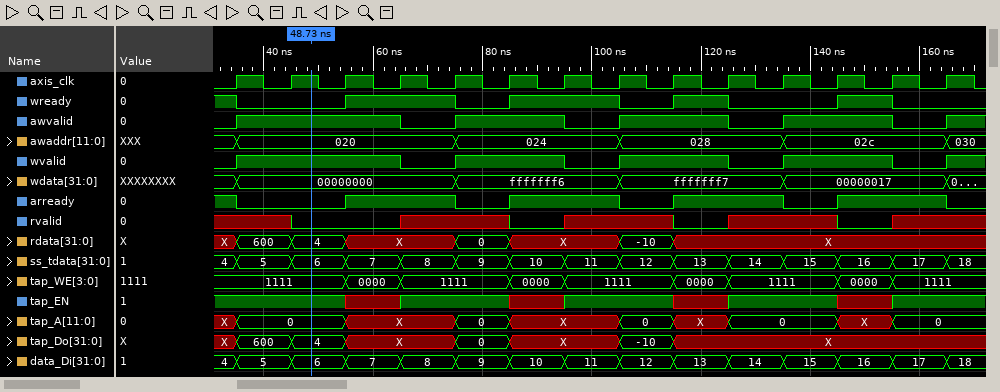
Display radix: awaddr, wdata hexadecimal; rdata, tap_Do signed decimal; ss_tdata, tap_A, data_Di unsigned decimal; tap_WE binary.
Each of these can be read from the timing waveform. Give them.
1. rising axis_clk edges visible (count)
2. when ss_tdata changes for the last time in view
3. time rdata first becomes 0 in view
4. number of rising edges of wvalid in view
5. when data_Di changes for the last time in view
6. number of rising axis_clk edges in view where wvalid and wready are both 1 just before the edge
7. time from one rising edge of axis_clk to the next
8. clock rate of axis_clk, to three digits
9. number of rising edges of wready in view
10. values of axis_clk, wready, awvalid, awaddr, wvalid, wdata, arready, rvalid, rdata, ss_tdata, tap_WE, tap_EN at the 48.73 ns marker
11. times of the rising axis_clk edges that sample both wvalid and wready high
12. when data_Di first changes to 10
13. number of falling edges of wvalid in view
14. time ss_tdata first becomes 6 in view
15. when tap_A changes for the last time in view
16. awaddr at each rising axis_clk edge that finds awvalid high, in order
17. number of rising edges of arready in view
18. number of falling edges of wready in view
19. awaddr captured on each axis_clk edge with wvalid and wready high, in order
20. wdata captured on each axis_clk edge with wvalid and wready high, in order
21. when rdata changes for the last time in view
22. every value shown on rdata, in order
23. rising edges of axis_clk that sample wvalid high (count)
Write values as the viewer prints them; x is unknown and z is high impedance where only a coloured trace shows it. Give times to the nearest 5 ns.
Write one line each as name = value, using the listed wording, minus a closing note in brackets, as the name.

rising axis_clk edges visible = 14
when ss_tdata changes for the last time in view = 165 ns
time rdata first becomes 0 in view = 75 ns
number of rising edges of wvalid in view = 5
when data_Di changes for the last time in view = 165 ns
number of rising axis_clk edges in view where wvalid and wready are both 1 just before the edge = 4
time from one rising edge of axis_clk to the next = 10 ns
clock rate of axis_clk, to three digits = 100 MHz
number of rising edges of wready in view = 4
values of axis_clk, wready, awvalid, awaddr, wvalid, wdata, arready, rvalid, rdata, ss_tdata, tap_WE, tap_EN at the 48.73 ns marker = axis_clk=1, wready=0, awvalid=1, awaddr=020, wvalid=1, wdata=00000000, arready=0, rvalid=0, rdata=4, ss_tdata=6, tap_WE=1111, tap_EN=1
times of the rising axis_clk edges that sample both wvalid and wready high = 65 ns, 95 ns, 125 ns, 155 ns
when data_Di first changes to 10 = 85 ns
number of falling edges of wvalid in view = 4
time ss_tdata first becomes 6 in view = 45 ns
when tap_A changes for the last time in view = 155 ns
awaddr at each rising axis_clk edge that finds awvalid high, in order = 020, 020, 020, 024, 024, 028, 028, 02c, 02c
number of rising edges of arready in view = 4
number of falling edges of wready in view = 5
awaddr captured on each axis_clk edge with wvalid and wready high, in order = 020, 024, 028, 02c
wdata captured on each axis_clk edge with wvalid and wready high, in order = 00000000, fffffff6, fffffff7, 00000017
when rdata changes for the last time in view = 115 ns
every value shown on rdata, in order = X, 600, 4, X, 0, X, -10, X
rising edges of axis_clk that sample wvalid high = 9
